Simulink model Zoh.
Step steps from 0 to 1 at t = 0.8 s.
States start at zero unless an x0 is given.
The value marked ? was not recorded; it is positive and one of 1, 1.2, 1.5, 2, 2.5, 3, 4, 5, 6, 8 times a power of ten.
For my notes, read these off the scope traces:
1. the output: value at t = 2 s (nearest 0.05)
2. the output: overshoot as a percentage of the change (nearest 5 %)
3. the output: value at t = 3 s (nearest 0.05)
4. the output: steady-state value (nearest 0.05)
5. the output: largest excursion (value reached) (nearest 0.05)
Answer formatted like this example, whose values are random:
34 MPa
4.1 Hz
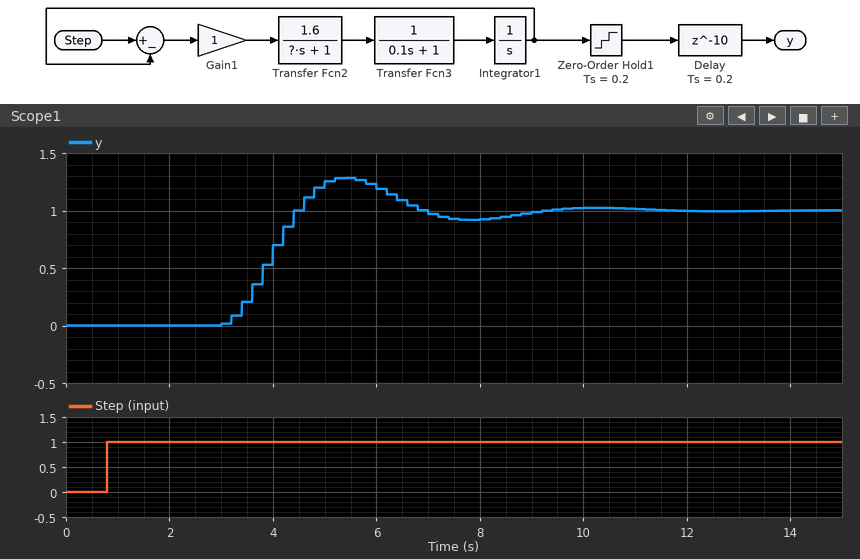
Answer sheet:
0.00
30 %
0.00
1.00
1.30
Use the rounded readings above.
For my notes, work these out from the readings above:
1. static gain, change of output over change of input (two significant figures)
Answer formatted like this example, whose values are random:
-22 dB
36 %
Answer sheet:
1.0
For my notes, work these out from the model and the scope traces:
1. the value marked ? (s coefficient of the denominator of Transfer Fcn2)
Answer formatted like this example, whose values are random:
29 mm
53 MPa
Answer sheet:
0.8
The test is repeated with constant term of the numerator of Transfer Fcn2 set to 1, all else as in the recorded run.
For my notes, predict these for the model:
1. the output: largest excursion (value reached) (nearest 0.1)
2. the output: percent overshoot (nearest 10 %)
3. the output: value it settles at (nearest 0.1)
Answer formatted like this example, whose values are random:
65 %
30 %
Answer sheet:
1.2
20 %
1.0
